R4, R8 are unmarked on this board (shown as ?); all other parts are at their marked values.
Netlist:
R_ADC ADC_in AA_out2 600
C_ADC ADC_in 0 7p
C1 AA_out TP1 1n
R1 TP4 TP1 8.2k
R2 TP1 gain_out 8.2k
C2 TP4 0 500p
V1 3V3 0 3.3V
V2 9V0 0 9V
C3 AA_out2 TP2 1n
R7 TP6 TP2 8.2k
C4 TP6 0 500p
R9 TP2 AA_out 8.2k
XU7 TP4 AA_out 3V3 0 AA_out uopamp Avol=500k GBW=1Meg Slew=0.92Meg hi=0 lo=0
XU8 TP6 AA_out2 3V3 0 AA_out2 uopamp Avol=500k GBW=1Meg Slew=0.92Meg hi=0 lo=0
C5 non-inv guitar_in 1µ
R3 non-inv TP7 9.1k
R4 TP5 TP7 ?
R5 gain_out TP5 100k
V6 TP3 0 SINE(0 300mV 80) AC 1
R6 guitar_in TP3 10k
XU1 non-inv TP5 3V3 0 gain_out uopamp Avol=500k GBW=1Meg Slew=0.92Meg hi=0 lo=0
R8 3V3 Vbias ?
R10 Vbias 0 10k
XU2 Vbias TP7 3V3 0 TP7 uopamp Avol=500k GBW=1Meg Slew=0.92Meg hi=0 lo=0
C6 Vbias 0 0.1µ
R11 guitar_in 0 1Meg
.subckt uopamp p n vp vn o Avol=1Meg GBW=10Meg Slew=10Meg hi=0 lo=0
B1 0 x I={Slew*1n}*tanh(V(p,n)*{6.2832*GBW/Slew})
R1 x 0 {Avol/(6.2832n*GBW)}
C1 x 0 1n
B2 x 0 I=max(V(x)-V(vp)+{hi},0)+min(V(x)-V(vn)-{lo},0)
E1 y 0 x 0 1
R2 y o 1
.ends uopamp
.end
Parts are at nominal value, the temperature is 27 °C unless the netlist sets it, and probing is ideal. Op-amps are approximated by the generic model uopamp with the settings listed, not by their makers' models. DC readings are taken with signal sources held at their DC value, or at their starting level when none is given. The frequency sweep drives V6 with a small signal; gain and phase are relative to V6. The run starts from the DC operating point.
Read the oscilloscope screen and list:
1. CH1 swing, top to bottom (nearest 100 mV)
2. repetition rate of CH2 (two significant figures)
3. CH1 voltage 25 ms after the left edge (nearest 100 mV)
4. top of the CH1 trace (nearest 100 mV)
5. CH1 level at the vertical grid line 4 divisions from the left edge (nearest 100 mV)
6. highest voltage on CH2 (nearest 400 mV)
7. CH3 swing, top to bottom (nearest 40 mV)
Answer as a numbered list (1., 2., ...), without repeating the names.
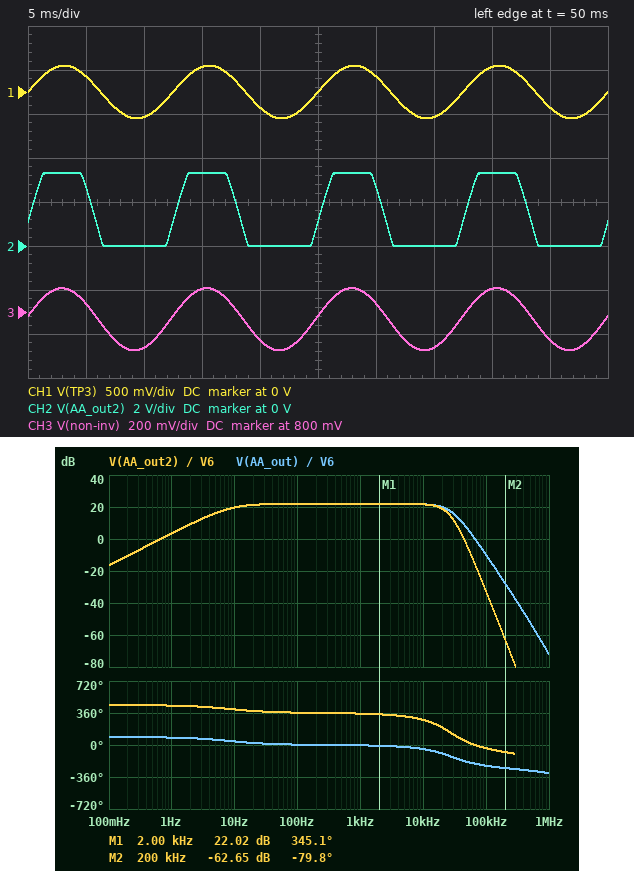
1. 600 mV
2. 80 Hz
3. 0 V
4. 300 mV
5. -200 mV
6. 3.2 V
7. 280 mV
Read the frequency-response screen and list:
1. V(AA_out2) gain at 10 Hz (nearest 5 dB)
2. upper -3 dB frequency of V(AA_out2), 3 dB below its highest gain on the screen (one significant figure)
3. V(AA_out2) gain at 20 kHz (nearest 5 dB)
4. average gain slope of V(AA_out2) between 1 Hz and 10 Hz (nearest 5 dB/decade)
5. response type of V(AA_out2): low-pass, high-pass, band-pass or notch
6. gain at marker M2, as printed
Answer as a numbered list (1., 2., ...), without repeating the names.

1. 20 dB
2. 20 kHz
3. 20 dB
4. 15 dB/decade
5. band-pass
6. -62.65 dB
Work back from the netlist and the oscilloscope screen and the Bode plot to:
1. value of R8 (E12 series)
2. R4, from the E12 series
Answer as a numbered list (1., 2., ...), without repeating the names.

1. 33 kΩ
2. 3.9 kΩ
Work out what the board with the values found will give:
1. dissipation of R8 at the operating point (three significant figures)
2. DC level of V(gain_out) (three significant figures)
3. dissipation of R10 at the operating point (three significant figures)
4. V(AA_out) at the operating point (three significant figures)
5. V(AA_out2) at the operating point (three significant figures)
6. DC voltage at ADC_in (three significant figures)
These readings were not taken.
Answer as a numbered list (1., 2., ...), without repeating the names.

1. 194 µW
2. 767 mV
3. 58.9 µW
4. 767 mV
5. 767 mV
6. 767 mV
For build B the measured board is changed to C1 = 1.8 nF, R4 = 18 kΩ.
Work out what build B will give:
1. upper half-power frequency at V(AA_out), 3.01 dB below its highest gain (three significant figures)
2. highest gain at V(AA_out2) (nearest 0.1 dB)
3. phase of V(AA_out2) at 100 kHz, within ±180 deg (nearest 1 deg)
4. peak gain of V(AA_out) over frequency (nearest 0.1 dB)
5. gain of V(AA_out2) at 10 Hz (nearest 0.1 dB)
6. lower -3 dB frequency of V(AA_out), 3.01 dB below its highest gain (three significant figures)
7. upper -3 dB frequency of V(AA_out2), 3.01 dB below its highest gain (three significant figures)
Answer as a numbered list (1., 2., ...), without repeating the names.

1. 23.2 kHz
2. 10.7 dB
3. -10 deg
4. 10.9 dB
5. 7.5 dB
6. 11.0 Hz
7. 21.2 kHz
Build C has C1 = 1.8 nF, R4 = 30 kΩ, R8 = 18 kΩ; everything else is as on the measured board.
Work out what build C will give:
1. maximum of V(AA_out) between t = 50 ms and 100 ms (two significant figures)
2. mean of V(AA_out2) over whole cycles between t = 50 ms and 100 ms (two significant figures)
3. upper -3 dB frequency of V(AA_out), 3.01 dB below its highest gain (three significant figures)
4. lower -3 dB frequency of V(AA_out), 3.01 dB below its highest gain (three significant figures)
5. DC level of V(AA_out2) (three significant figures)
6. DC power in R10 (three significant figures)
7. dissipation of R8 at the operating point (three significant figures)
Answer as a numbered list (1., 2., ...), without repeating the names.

1. 1.8 V
2. 1.2 V
3. 23.3 kHz
4. 11.1 Hz
5. 1.18 V
6. 139 µW
7. 250 µW
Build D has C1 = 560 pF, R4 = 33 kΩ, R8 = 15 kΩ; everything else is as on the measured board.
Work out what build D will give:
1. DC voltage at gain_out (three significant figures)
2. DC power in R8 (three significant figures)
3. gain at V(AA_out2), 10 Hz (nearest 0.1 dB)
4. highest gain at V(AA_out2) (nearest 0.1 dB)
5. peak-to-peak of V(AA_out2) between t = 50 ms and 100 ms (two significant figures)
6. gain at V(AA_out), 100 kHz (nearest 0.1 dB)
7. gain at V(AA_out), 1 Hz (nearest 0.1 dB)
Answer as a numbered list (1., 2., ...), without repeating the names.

1. 1.32 V
2. 261 µW
3. 3.3 dB
4. 5.6 dB
5. 1.1 V
6. -13.6 dB
7. -12.9 dB
